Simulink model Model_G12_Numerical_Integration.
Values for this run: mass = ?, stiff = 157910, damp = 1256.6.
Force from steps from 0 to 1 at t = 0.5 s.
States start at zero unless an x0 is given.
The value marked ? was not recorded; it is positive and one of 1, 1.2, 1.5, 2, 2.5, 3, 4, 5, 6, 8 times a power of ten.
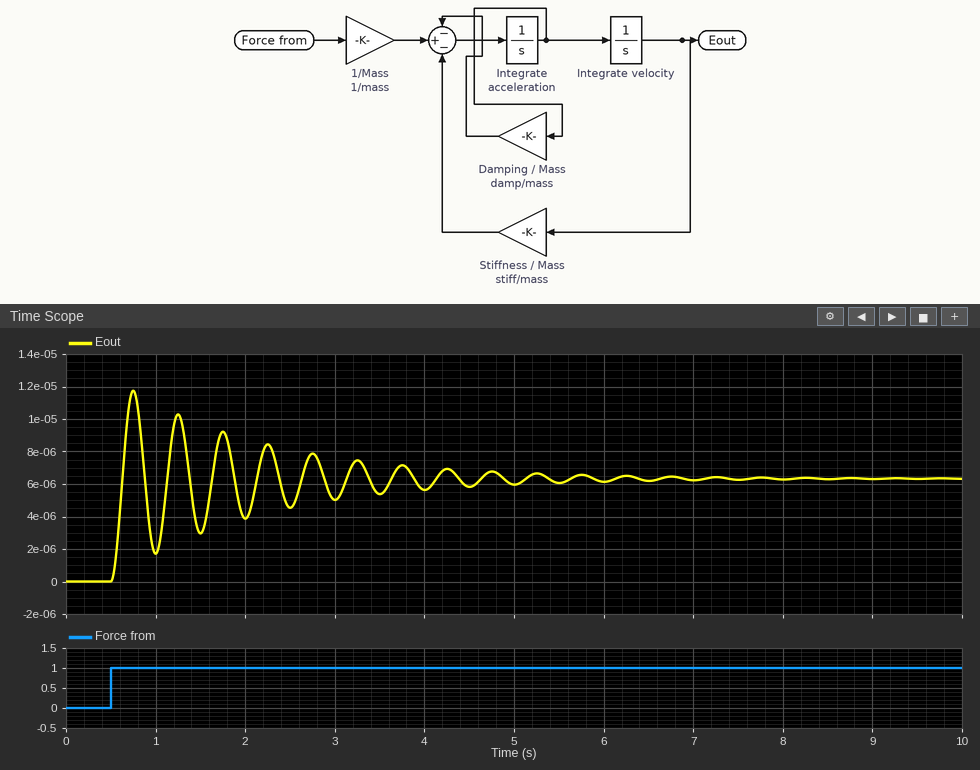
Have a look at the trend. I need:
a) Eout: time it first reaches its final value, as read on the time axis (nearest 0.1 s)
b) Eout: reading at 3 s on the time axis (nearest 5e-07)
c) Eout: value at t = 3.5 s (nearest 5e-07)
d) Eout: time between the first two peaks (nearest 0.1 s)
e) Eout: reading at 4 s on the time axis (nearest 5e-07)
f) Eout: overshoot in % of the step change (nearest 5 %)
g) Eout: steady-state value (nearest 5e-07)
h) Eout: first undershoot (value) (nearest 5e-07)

0.6 s
0.0000050
0.0000055
0.5 s
0.0000055
85 %
0.0000065
0.0000015
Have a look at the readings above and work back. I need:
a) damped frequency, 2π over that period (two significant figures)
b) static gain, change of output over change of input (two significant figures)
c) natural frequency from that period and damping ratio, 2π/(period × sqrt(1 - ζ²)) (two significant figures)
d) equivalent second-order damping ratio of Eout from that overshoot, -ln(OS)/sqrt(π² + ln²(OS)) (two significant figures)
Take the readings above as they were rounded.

13 rad/s
0.0000065
13 rad/s
0.052
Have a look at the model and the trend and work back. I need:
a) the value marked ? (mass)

1000
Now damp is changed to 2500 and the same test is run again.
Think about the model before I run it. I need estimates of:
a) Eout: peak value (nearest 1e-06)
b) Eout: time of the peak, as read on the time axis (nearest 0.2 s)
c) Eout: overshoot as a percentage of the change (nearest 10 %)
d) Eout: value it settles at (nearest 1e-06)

0.000011
0.8 s
70 %
0.000006
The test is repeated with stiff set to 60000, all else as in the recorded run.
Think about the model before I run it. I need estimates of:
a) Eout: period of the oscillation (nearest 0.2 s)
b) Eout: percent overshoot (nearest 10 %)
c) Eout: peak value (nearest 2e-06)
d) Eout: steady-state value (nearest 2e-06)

0.8 s
80 %
0.000030
0.000016
